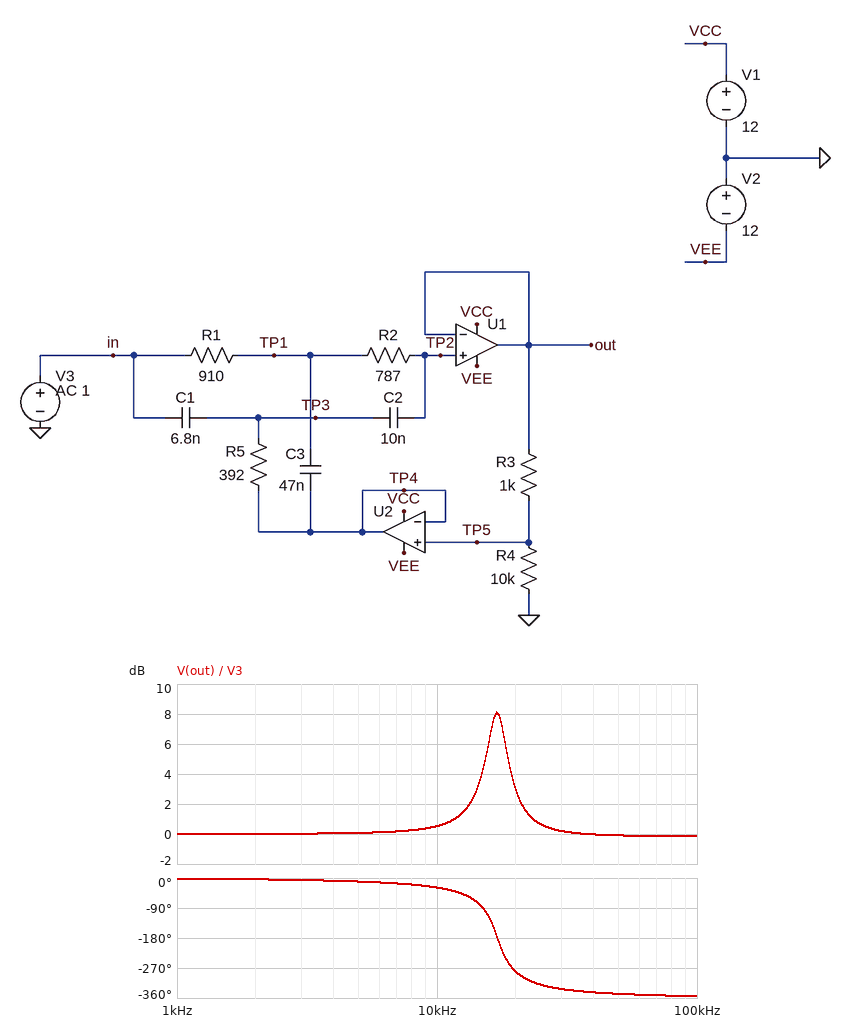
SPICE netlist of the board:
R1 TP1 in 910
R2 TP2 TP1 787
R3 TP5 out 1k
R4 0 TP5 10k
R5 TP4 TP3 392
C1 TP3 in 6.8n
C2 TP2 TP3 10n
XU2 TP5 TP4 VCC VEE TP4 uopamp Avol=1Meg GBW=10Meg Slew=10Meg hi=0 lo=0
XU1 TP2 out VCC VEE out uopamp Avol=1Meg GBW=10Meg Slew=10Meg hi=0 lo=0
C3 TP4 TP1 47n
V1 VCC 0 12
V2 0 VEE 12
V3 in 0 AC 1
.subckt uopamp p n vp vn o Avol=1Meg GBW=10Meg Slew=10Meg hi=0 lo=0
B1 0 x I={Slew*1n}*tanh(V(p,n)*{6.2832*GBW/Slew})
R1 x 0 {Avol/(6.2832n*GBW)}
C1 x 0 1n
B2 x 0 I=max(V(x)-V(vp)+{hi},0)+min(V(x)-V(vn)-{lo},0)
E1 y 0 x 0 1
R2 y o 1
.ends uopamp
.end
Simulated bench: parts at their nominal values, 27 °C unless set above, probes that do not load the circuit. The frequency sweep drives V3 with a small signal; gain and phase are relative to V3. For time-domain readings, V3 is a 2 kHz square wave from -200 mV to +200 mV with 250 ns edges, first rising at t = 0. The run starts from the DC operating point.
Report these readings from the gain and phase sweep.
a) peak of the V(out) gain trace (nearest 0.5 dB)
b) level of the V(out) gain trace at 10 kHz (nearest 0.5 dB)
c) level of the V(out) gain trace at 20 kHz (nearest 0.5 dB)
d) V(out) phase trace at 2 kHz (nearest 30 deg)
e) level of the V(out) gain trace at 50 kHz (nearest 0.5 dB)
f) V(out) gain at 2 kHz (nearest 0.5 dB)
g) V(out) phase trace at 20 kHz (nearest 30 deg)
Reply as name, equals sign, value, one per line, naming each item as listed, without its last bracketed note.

peak of the V(out) gain trace = 8.0 dB
level of the V(out) gain trace at 10 kHz = 0.5 dB
level of the V(out) gain trace at 20 kHz = 3.0 dB
V(out) phase trace at 2 kHz = 0 deg
level of the V(out) gain trace at 50 kHz = 0 dB
V(out) gain at 2 kHz = 0 dB
V(out) phase trace at 20 kHz = -270 deg
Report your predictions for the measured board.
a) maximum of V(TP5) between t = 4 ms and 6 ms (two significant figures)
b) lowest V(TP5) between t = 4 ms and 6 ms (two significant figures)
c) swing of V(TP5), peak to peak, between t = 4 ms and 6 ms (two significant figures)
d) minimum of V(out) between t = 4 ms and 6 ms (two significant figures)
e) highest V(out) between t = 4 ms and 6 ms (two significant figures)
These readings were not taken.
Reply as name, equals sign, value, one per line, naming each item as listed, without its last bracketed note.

maximum of V(TP5) between t = 4 ms and 6 ms = 320 mV
lowest V(TP5) between t = 4 ms and 6 ms = -320 mV
swing of V(TP5), peak to peak, between t = 4 ms and 6 ms = 640 mV
minimum of V(out) between t = 4 ms and 6 ms = -350 mV
highest V(out) between t = 4 ms and 6 ms = 350 mV
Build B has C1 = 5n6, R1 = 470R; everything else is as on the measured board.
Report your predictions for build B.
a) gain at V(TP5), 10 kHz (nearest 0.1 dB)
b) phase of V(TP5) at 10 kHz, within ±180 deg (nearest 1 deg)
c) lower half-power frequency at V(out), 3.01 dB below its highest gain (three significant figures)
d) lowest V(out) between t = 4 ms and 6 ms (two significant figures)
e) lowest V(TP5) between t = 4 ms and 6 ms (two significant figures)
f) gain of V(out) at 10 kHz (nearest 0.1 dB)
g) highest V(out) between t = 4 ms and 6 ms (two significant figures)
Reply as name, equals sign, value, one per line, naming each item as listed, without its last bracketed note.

gain at V(TP5), 10 kHz = -0.6 dB
phase of V(TP5) at 10 kHz, within ±180 deg = -14 deg
lower half-power frequency at V(out), 3.01 dB below its highest gain = 20.3 kHz
lowest V(out) between t = 4 ms and 6 ms = -340 mV
lowest V(TP5) between t = 4 ms and 6 ms = -310 mV
gain of V(out) at 10 kHz = 0.2 dB
highest V(out) between t = 4 ms and 6 ms = 340 mV
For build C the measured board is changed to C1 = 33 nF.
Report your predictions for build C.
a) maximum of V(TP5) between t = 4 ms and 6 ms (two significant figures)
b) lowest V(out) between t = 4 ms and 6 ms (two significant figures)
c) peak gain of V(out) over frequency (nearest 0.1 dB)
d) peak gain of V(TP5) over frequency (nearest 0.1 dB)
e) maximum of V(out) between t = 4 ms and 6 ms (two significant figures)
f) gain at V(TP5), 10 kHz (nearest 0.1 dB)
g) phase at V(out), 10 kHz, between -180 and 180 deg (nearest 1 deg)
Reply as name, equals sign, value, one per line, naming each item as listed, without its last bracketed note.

maximum of V(TP5) between t = 4 ms and 6 ms = 260 mV
lowest V(out) between t = 4 ms and 6 ms = -280 mV
peak gain of V(out) over frequency = 0 dB
peak gain of V(TP5) over frequency = -0.8 dB
maximum of V(out) between t = 4 ms and 6 ms = 280 mV
gain at V(TP5), 10 kHz = -10.3 dB
phase at V(out), 10 kHz, between -180 and 180 deg = -138 deg
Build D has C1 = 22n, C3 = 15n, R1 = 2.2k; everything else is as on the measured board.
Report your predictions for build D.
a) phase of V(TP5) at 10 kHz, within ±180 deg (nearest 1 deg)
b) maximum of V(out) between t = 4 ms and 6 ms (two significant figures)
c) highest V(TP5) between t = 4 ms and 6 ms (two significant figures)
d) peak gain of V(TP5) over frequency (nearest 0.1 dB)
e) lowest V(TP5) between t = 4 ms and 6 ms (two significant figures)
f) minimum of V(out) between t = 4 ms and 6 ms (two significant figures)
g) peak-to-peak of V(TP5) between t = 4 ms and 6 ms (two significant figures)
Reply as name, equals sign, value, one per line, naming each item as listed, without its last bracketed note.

phase of V(TP5) at 10 kHz, within ±180 deg = -20 deg
maximum of V(out) between t = 4 ms and 6 ms = 240 mV
highest V(TP5) between t = 4 ms and 6 ms = 220 mV
peak gain of V(TP5) over frequency = -0.8 dB
lowest V(TP5) between t = 4 ms and 6 ms = -220 mV
minimum of V(out) between t = 4 ms and 6 ms = -240 mV
peak-to-peak of V(TP5) between t = 4 ms and 6 ms = 440 mV
